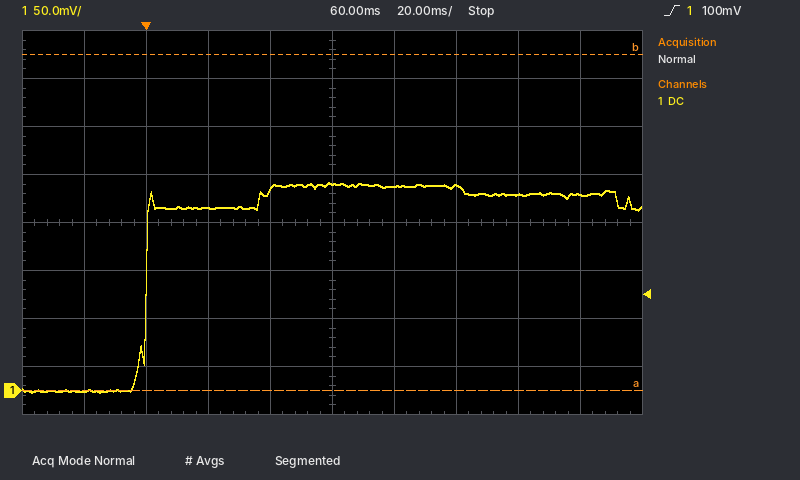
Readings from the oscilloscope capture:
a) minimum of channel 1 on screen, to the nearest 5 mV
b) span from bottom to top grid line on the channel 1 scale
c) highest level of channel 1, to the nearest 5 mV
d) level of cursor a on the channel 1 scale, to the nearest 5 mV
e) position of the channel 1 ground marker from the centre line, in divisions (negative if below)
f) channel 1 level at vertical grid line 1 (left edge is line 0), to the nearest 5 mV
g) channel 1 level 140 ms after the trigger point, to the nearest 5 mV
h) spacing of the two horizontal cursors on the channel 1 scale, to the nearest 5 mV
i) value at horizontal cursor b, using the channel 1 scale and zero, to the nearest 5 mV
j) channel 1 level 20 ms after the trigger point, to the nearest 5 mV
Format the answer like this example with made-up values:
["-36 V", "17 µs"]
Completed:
["0 mV", "400 mV", "215 mV", "0 mV", "-3.5 div", "0 mV", "205 mV", "350 mV", "350 mV", "190 mV"]
